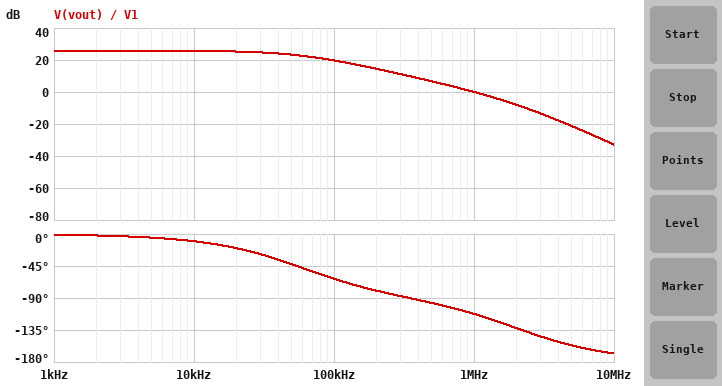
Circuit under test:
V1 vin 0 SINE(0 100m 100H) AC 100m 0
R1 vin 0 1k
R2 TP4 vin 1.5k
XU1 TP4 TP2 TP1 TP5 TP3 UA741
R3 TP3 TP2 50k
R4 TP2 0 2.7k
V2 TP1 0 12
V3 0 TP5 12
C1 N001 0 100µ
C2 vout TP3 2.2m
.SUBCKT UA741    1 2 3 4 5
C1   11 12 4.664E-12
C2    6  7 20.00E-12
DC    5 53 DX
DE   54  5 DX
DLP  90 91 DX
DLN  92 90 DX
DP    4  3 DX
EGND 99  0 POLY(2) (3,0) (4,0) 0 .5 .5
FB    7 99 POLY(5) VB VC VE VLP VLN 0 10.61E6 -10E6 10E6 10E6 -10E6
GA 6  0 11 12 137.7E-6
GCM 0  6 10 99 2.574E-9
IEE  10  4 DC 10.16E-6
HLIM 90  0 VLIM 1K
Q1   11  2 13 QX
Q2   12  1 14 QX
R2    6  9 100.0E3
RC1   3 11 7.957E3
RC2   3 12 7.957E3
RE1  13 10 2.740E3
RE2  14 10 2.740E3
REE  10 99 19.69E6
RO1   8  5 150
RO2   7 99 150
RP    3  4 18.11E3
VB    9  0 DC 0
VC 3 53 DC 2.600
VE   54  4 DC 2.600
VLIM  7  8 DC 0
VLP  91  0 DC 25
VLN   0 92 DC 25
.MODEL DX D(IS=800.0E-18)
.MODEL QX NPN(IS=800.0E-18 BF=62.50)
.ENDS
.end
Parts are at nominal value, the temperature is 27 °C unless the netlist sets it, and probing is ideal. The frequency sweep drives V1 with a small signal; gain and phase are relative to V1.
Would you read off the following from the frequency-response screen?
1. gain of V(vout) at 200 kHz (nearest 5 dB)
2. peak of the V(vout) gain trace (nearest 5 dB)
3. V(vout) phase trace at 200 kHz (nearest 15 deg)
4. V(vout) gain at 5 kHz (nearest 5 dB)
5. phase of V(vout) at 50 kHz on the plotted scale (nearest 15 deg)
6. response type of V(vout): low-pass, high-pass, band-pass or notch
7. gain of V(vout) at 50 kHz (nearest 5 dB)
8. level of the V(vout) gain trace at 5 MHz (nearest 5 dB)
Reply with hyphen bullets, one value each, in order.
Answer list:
- 15 dB
- 25 dB
- -75 deg
- 25 dB
- -45 deg
- low-pass
- 25 dB
- -20 dB
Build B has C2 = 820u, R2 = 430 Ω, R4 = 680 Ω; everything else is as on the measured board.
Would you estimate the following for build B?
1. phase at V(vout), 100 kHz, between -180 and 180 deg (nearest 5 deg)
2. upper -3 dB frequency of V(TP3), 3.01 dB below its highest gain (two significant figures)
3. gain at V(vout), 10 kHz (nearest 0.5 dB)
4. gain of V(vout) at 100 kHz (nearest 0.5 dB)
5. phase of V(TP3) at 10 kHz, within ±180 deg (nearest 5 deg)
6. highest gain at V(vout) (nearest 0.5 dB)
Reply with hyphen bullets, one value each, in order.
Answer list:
- -85 deg
- 15 kHz
- 36.0 dB
- 20.5 dB
- -35 deg
- 37.5 dB
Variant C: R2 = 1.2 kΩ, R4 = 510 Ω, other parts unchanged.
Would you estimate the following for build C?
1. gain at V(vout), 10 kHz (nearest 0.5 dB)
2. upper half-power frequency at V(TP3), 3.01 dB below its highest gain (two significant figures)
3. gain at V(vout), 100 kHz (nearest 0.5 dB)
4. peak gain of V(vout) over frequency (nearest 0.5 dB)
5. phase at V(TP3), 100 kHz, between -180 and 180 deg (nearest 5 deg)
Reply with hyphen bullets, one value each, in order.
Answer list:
- 37.5 dB
- 11 kHz
- 20.5 dB
- 40.0 dB
- -85 deg
